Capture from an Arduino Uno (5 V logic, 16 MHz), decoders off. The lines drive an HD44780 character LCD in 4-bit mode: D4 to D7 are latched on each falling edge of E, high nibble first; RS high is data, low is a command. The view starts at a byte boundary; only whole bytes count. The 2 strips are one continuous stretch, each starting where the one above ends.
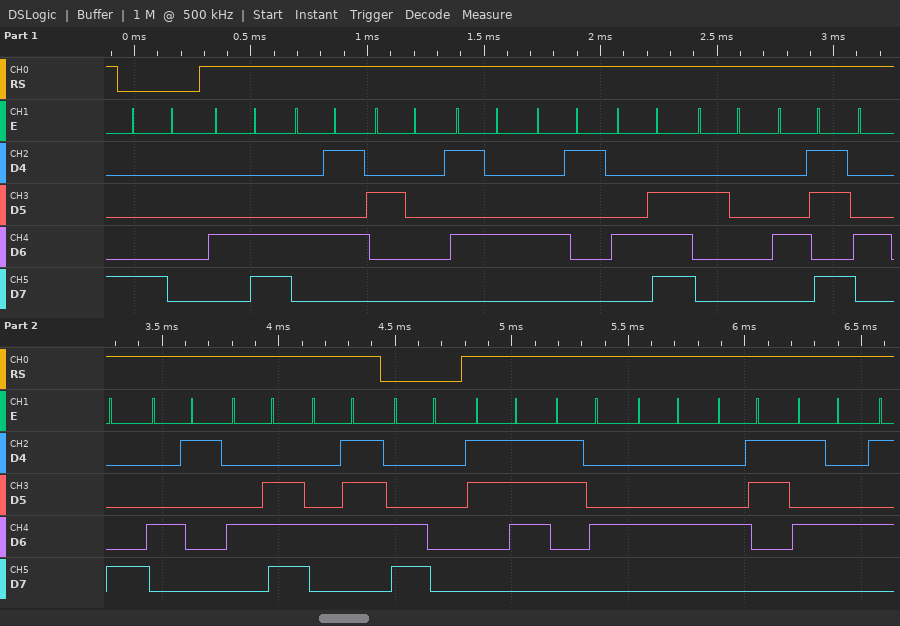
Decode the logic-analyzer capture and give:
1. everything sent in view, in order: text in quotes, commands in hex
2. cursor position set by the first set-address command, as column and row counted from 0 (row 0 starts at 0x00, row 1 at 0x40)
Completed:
0x80 "LE TAN KHANG" 0xC0 "74DCT"
column 0, row 0
